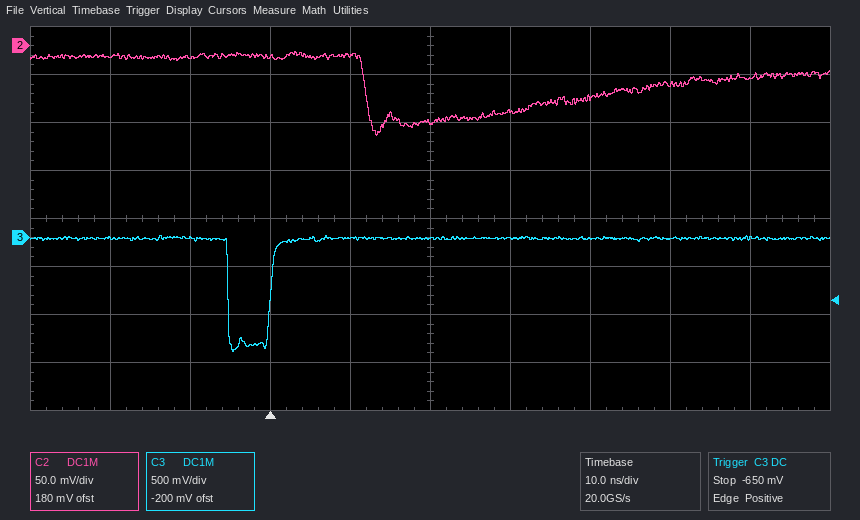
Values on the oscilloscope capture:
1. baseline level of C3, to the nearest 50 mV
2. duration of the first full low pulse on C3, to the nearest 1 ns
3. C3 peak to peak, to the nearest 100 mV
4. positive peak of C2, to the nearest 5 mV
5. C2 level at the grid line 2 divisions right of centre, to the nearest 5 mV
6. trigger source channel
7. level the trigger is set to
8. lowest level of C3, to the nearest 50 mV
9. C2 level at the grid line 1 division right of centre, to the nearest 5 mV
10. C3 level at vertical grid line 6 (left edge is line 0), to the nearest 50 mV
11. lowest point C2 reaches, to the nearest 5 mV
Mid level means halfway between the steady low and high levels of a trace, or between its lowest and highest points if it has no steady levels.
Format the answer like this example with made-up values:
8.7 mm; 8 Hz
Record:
0 mV; 5 ns; 1.20 V; -5 mV; -55 mV; C3; -650 mV; -1.20 V; -70 mV; 0 mV; -95 mV
